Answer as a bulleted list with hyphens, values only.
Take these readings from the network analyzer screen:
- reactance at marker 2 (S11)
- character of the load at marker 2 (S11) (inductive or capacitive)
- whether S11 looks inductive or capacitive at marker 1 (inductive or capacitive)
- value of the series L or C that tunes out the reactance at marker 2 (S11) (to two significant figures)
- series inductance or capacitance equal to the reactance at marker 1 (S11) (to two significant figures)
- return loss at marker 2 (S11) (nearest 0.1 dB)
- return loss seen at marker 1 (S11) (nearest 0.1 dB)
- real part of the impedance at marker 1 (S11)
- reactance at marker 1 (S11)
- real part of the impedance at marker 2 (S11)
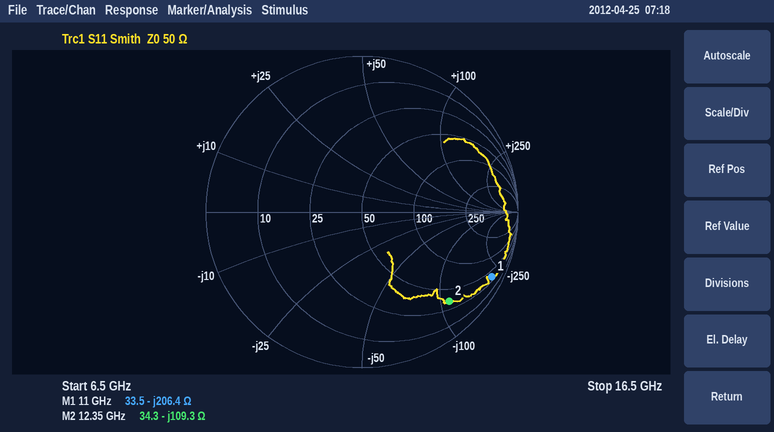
- -109.3 Ω
- capacitive
- capacitive
- 1.4 nH
- 70 fF
- 1.9 dB
- 0.6 dB
- 33.5 Ω
- -206.4 Ω
- 34.3 Ω
